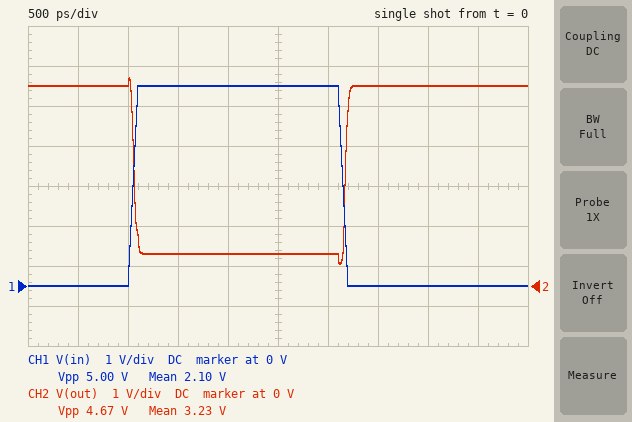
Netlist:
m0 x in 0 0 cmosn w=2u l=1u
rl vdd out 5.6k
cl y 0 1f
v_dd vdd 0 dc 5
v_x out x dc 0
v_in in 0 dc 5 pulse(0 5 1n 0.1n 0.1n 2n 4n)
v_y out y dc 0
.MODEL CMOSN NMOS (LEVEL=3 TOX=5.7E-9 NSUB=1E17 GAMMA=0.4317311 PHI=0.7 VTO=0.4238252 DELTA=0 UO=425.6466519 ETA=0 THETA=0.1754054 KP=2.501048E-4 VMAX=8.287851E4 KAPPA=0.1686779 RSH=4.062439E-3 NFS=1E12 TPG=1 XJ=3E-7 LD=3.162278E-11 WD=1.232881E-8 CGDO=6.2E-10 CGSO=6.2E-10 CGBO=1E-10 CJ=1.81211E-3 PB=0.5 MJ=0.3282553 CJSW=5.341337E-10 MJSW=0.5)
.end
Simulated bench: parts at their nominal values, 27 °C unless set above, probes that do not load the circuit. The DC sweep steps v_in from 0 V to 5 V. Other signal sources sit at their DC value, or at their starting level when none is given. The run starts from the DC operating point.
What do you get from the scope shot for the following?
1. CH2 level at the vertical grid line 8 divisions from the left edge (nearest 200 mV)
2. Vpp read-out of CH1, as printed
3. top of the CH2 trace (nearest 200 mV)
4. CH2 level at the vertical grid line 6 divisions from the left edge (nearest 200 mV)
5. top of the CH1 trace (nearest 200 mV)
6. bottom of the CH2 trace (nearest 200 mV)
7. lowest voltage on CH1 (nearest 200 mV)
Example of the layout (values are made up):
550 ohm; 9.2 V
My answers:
5.0 V; 5.00 V; 5.2 V; 800 mV; 5.0 V; 600 mV; 0 V
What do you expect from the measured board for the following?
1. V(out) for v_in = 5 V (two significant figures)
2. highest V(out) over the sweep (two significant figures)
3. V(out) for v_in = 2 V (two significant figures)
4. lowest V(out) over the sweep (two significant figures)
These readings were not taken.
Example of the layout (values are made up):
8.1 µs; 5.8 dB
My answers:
810 mV; 5.0 V; 3.3 V; 810 mV
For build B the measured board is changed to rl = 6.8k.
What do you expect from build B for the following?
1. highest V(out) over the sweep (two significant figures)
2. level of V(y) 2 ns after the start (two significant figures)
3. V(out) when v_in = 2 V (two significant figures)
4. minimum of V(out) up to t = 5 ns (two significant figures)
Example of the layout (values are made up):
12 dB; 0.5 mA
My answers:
5.0 V; 650 mV; 2.9 V; 380 mV
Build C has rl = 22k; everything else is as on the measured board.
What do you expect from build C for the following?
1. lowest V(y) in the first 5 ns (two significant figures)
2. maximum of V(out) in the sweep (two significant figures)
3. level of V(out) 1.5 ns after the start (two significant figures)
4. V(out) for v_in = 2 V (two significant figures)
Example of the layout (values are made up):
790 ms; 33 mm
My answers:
-580 mV; 5.0 V; 190 mV; 470 mV
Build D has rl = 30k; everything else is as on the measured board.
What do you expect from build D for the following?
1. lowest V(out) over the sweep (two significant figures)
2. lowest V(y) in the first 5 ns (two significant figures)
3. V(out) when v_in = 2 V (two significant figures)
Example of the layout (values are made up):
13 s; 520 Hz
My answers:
140 mV; -620 mV; 320 mV
